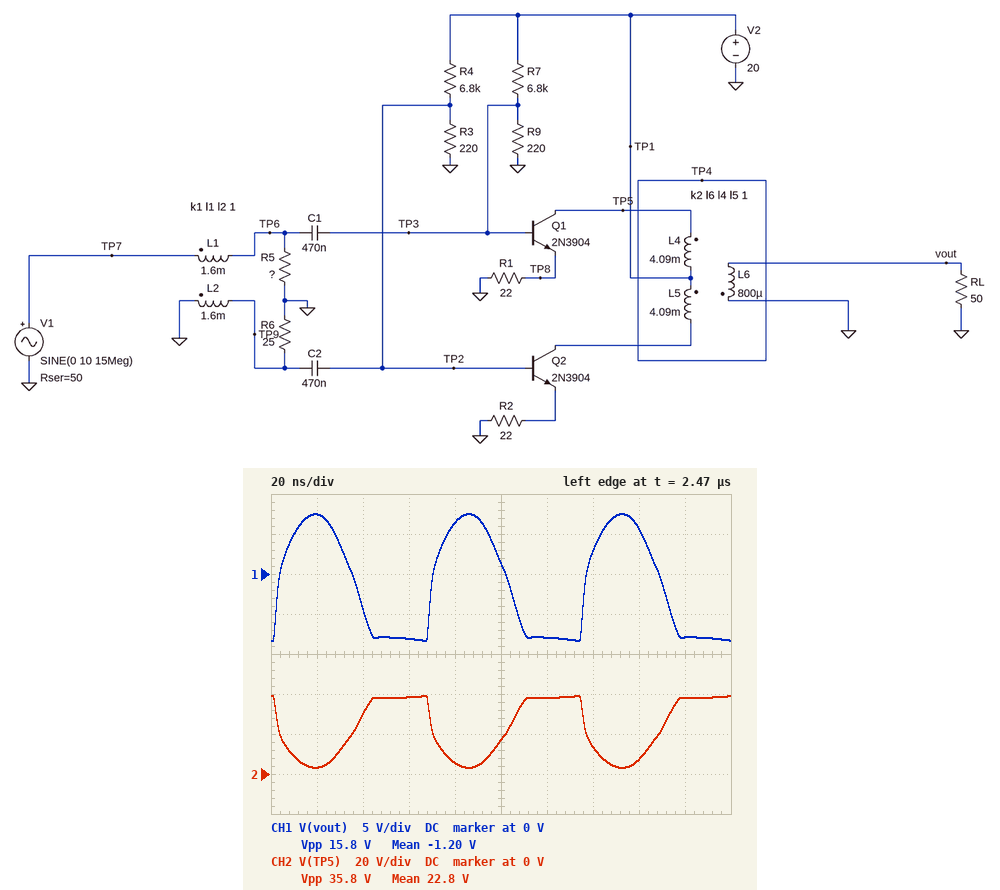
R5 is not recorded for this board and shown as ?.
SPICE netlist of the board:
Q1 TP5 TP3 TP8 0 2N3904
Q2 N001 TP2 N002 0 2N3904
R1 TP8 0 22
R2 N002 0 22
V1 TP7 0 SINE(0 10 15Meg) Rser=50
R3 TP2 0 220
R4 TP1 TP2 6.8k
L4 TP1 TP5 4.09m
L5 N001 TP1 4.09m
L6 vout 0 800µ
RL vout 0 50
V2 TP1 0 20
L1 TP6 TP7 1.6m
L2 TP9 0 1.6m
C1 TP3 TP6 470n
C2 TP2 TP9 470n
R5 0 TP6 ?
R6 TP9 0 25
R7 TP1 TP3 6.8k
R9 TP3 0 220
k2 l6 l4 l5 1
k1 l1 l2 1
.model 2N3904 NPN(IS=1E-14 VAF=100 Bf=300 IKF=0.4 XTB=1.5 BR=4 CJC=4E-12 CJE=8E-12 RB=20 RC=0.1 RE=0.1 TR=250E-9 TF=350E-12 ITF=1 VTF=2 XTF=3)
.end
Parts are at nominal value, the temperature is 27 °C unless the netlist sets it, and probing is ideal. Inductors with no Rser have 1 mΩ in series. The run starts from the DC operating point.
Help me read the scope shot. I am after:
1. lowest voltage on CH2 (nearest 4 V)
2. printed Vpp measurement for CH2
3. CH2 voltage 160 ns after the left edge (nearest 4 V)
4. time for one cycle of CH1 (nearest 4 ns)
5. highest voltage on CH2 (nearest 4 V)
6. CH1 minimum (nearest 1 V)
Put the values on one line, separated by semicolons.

4 V; 35.8 V; 8 V; 68 ns; 40 V; -8 V
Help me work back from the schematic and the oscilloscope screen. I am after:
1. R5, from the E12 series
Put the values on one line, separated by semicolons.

15 Ω
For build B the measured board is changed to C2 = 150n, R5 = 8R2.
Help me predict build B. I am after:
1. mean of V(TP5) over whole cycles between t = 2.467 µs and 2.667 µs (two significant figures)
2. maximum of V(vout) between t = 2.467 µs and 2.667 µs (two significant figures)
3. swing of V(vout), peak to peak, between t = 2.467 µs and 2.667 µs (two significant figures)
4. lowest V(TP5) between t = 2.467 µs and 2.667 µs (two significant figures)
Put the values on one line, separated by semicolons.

25 V; 4.7 V; 13 V; 9.4 V
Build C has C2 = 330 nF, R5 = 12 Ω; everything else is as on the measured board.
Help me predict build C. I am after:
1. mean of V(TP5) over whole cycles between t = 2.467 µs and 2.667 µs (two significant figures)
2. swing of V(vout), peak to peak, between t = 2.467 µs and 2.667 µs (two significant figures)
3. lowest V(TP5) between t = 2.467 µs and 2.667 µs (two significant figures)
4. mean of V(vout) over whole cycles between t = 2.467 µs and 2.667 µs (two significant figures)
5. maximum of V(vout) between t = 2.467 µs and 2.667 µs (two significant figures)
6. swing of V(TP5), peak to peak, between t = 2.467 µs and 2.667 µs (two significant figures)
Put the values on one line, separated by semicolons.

24 V; 15 V; 5.6 V; -1.6 V; 6.4 V; 33 V
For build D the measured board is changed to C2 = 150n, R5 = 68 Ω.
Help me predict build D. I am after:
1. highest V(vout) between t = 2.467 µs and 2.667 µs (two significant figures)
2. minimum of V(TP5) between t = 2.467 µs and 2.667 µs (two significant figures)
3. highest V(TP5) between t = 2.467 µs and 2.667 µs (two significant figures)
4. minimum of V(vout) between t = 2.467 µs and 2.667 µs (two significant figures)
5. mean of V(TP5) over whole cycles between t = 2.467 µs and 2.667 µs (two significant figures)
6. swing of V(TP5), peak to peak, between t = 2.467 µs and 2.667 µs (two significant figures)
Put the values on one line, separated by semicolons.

8.3 V; 1.2 V; 38 V; -8.1 V; 16 V; 37 V
